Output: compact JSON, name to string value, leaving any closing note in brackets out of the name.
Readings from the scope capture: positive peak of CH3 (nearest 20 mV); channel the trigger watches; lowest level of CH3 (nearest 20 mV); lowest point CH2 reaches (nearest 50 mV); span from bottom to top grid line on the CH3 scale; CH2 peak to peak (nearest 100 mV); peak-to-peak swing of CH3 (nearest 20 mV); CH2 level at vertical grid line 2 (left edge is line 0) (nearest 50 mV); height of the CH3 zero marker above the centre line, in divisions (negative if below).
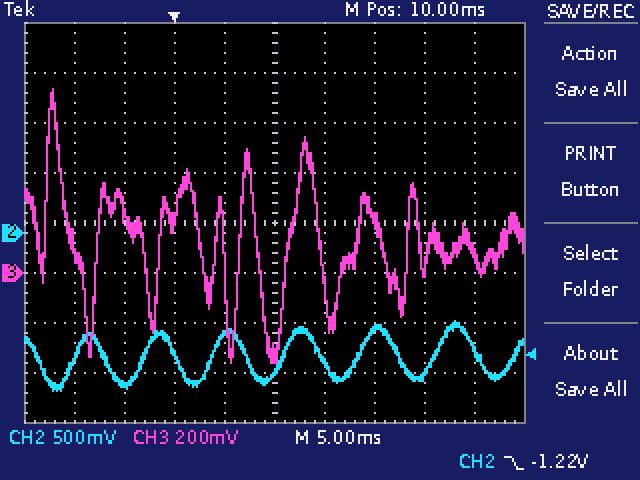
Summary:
{"positive peak of CH3": "740 mV", "channel the trigger watches": "CH2", "lowest level of CH3": "-360 mV", "lowest point CH2 reaches": "-1.60 V", "span from bottom to top grid line on the CH3 scale": "1.6 V", "CH2 peak to peak": "700 mV", "peak-to-peak swing of CH3": "1.10 V", "CH2 level at vertical grid line 2 (left edge is line 0)": "-1.50 V", "height of the CH3 zero marker above the centre line, in divisions": "-1.0 div"}
